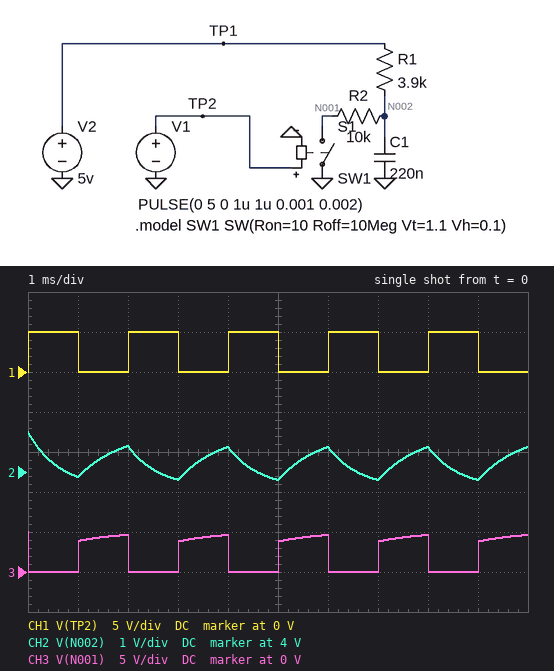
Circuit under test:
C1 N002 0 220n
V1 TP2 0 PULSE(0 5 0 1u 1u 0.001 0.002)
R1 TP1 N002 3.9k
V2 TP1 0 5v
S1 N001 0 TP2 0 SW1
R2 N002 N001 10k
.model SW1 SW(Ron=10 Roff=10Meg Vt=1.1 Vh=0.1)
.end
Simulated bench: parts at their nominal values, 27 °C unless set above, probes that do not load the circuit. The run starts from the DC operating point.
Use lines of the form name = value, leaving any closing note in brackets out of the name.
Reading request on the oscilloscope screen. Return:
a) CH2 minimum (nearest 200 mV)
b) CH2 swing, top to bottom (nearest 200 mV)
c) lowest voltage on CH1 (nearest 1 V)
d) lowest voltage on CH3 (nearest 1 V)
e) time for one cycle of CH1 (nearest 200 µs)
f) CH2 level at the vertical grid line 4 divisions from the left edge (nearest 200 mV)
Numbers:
CH2 minimum = 3.8 V
CH2 swing, top to bottom = 1.2 V
lowest voltage on CH1 = 0 V
lowest voltage on CH3 = 0 V
time for one cycle of CH1 = 2.0 ms
CH2 level at the vertical grid line 4 divisions from the left edge = 4.6 V
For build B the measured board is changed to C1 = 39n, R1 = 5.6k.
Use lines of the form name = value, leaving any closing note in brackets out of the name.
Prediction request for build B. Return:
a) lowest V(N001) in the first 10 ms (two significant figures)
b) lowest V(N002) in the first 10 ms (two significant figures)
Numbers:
lowest V(N001) in the first 10 ms = 3.2 mV
lowest V(N002) in the first 10 ms = 3.2 V
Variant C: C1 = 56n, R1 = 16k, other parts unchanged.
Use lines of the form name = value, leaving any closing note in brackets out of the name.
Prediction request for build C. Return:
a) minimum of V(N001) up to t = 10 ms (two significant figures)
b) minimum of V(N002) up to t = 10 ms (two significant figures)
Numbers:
minimum of V(N001) up to t = 10 ms = 2.0 mV
minimum of V(N002) up to t = 10 ms = 2.0 V
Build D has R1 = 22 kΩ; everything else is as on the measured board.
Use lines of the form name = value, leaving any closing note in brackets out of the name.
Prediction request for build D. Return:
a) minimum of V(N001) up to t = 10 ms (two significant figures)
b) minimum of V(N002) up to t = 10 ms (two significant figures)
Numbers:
minimum of V(N001) up to t = 10 ms = 2.2 mV
minimum of V(N002) up to t = 10 ms = 2.2 V
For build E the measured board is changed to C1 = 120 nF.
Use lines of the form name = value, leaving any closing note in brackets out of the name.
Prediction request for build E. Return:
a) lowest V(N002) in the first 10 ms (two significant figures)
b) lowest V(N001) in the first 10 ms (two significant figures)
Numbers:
lowest V(N002) in the first 10 ms = 3.7 V
lowest V(N001) in the first 10 ms = 3.7 mV
